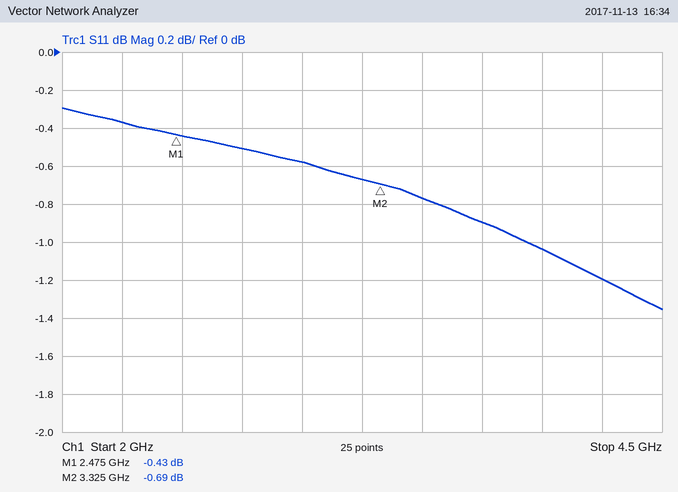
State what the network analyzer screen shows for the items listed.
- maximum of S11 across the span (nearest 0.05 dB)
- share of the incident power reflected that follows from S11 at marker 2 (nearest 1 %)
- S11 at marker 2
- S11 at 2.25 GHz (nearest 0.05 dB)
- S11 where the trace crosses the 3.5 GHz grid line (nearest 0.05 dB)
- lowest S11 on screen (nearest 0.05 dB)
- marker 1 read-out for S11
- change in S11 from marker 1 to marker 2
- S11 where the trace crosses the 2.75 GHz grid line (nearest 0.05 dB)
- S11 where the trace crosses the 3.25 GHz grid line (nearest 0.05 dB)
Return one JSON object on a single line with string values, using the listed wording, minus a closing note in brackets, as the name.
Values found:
{"maximum of S11 across the span": "-0.30 dB", "share of the incident power reflected that follows from S11 at marker 2": "85 %", "S11 at marker 2": "-0.69 dB", "S11 at 2.25 GHz": "-0.35 dB", "S11 where the trace crosses the 3.5 GHz grid line": "-0.75 dB", "lowest S11 on screen": "-1.35 dB", "marker 1 read-out for S11": "-0.43 dB", "change in S11 from marker 1 to marker 2": "-0.26 dB", "S11 where the trace crosses the 2.75 GHz grid line": "-0.50 dB", "S11 where the trace crosses the 3.25 GHz grid line": "-0.65 dB"}
